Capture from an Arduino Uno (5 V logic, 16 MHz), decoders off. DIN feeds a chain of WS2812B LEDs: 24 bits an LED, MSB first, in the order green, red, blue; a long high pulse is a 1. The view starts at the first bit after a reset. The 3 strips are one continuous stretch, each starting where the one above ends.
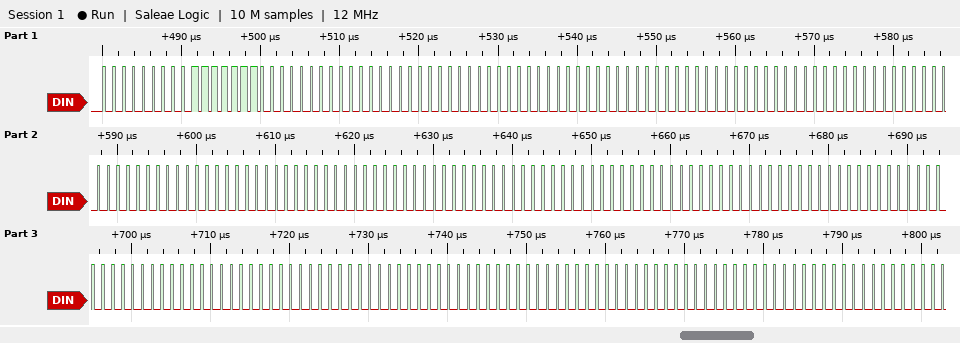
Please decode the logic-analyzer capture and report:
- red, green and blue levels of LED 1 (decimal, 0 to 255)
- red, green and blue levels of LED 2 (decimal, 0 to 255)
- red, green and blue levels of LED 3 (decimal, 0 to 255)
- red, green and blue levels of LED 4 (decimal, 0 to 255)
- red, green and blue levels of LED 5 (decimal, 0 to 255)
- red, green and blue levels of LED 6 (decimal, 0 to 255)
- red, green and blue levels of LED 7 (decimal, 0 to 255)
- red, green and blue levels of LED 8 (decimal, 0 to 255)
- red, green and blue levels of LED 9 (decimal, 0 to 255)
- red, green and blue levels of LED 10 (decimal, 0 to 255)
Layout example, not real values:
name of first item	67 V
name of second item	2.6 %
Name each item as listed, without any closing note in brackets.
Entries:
red, green and blue levels of LED 1	127, 0, 0
red, green and blue levels of LED 2	0, 0, 0
red, green and blue levels of LED 3	0, 0, 0
red, green and blue levels of LED 4	0, 0, 0
red, green and blue levels of LED 5	0, 0, 0
red, green and blue levels of LED 6	0, 0, 0
red, green and blue levels of LED 7	0, 0, 0
red, green and blue levels of LED 8	0, 0, 0
red, green and blue levels of LED 9	0, 0, 0
red, green and blue levels of LED 10	0, 0, 0
